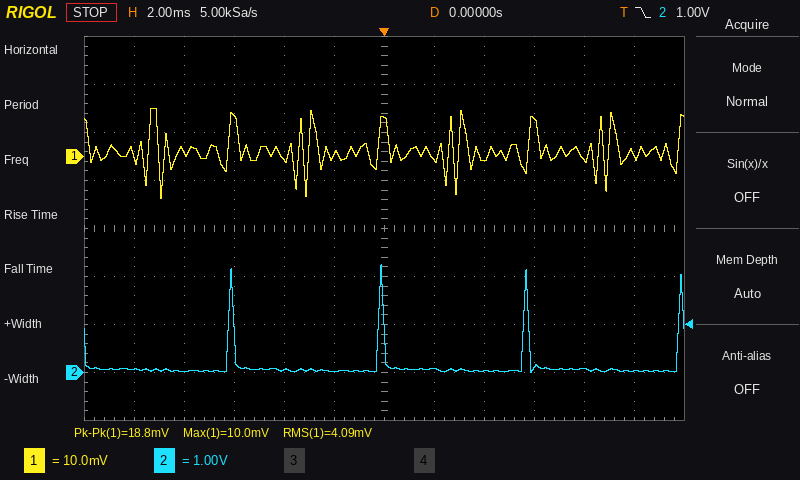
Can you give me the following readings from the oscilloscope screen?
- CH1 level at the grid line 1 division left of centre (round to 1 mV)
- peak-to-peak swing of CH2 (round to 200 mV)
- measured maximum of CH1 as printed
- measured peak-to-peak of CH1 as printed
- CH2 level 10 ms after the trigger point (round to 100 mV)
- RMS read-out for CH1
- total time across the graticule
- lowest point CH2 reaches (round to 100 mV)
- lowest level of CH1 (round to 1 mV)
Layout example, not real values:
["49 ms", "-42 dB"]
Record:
["0 mV", "2.2 V", "10.0 mV", "18.8 mV", "0.0 V", "4.09 mV", "24 ms", "0.0 V", "-9 mV"]
